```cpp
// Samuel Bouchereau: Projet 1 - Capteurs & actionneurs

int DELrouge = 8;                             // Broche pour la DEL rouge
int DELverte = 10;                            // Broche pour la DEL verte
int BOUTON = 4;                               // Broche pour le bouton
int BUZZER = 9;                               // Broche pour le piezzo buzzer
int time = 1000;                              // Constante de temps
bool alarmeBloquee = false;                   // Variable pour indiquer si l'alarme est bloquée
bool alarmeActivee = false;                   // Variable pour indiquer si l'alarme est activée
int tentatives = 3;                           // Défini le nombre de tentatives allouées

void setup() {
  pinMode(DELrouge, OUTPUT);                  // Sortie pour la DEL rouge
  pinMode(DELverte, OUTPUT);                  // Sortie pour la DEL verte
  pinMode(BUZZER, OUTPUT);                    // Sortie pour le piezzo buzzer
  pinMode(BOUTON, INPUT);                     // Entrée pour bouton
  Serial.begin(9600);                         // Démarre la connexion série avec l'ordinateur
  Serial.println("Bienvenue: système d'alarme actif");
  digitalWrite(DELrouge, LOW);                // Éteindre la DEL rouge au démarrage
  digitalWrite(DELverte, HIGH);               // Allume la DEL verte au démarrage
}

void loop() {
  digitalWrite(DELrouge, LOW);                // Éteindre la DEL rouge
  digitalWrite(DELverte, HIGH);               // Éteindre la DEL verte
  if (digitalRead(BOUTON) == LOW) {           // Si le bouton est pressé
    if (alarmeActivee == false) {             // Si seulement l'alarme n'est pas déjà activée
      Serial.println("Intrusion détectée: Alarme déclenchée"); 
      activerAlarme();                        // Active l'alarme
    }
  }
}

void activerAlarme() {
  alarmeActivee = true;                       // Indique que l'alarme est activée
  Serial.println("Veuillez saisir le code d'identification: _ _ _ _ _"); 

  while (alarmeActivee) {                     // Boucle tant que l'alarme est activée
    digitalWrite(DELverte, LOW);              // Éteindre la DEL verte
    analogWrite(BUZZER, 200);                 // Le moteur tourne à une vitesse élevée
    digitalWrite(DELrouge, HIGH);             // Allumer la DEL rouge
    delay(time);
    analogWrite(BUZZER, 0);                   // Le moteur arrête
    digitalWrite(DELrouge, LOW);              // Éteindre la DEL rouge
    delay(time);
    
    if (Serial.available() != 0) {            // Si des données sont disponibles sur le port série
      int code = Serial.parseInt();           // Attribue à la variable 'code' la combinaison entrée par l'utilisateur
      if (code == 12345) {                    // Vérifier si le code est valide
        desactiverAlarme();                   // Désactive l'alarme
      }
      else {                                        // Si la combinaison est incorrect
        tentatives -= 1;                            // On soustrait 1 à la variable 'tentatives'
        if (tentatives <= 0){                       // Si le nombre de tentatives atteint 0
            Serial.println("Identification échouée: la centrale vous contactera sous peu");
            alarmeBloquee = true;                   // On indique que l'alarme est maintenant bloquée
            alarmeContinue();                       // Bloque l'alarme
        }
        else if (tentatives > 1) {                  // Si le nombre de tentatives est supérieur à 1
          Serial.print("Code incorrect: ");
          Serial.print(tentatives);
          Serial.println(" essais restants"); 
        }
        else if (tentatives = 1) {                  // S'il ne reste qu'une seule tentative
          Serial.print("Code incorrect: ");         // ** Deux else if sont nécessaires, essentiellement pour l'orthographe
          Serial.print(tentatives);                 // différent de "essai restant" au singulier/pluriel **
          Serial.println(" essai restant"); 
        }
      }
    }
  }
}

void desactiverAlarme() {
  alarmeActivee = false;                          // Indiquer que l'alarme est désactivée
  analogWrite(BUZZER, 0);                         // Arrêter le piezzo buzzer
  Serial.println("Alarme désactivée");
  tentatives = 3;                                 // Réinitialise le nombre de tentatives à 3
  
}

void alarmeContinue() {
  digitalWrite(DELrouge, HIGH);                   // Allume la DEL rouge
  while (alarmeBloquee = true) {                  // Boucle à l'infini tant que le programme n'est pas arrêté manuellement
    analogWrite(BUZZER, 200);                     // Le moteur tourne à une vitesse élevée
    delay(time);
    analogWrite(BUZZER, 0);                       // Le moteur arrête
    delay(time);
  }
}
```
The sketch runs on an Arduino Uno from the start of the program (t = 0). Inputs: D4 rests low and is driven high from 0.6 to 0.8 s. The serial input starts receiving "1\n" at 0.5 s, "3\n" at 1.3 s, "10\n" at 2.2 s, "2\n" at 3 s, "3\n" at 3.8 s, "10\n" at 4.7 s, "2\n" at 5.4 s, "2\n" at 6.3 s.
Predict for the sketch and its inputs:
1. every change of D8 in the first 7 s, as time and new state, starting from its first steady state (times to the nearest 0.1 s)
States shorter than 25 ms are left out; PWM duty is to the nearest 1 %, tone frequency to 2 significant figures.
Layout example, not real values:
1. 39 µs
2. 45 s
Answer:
1. 0 s low; 0.1 s high; 1.1 s low; 2.1 s high; 3.1 s low; 4.1 s high; 5.1 s low; 6.1 s high
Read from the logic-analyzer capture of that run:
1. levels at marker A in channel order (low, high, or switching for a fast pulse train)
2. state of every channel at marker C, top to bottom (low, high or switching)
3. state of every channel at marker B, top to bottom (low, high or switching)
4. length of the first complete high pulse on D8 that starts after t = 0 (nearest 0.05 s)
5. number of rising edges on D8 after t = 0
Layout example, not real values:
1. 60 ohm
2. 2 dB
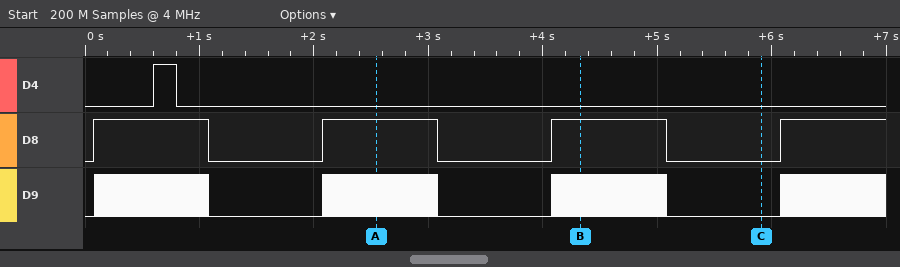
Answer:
1. D4 low, D8 high, D9 switching
2. D4 low, D8 low, D9 low
3. D4 low, D8 high, D9 switching
4. 1.00 s
5. 4
